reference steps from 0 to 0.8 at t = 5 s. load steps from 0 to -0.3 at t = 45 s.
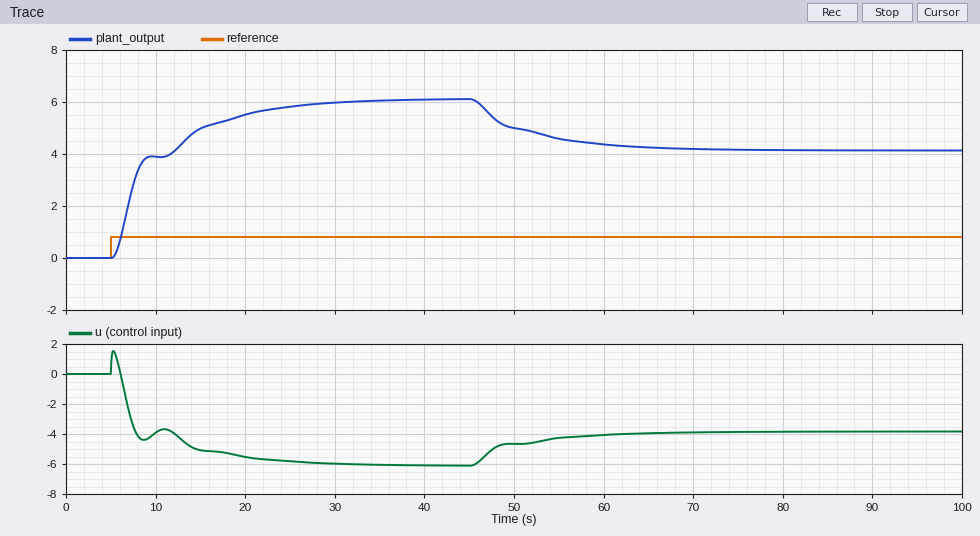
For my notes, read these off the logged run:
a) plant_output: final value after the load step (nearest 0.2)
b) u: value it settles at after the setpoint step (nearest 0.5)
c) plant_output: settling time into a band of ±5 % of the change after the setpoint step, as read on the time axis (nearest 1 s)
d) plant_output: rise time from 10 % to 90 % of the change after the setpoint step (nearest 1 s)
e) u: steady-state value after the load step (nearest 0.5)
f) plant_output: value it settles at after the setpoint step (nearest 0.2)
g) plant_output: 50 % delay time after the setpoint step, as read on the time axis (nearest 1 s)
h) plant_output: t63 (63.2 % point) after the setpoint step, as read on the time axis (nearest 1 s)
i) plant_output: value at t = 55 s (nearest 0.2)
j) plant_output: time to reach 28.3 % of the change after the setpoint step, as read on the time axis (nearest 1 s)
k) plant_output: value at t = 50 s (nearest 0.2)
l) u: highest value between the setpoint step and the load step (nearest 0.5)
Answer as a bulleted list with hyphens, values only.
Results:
- 4.2
- -6.0
- 25 s
- 14 s
- -4.0
- 6.2
- 8 s
- 9 s
- 4.6
- 7 s
- 5.0
- 1.5
